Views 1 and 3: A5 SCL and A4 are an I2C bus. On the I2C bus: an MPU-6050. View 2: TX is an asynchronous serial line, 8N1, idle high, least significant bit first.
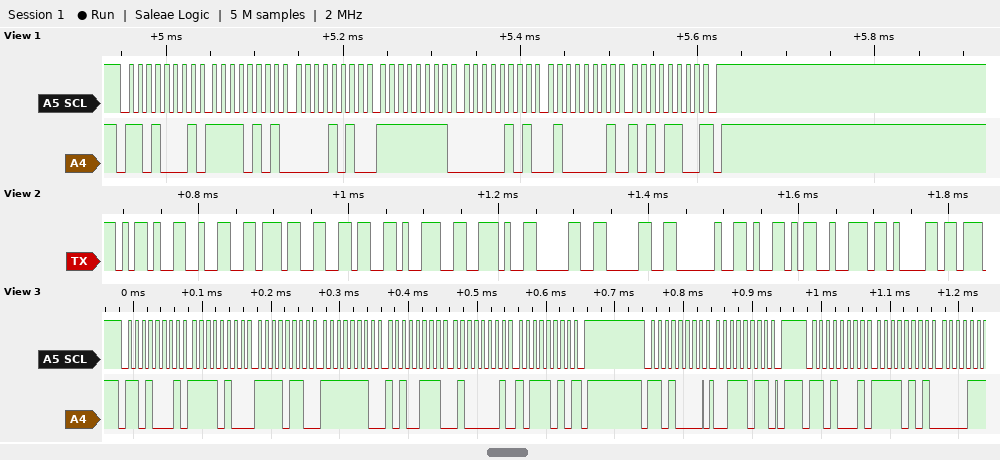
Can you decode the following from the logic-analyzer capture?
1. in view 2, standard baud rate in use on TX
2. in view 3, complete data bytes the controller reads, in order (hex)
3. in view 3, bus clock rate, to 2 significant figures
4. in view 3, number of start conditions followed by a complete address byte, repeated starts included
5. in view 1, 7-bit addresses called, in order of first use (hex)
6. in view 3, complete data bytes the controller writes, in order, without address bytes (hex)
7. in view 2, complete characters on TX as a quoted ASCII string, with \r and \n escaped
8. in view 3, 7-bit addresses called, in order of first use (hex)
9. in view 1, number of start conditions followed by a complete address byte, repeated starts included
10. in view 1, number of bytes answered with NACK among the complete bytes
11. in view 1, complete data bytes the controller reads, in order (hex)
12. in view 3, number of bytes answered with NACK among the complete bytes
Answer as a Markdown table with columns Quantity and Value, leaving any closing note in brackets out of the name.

| Quantity | Value |
|---|---|
| in view 2, standard baud rate in use on TX | 115200 baud |
| in view 3, complete data bytes the controller reads, in order | F4 F6 FE A7 41 BA F5 |
| in view 3, bus clock rate, to 2 significant figures | 100 kHz |
| in view 3, number of start conditions followed by a complete address byte, repeated starts included | 3 |
| in view 1, 7-bit addresses called, in order of first use | 0x68 |
| in view 3, complete data bytes the controller writes, in order, without address bytes | 3B |
| in view 2, complete characters on TX as a quoted ASCII string, with \r and \n escaped | "-2769.00 Yra" |
| in view 3, 7-bit addresses called, in order of first use | 0x68 |
| in view 1, number of start conditions followed by a complete address byte, repeated starts included | 1 |
| in view 1, number of bytes answered with NACK among the complete bytes | 1 |
| in view 1, complete data bytes the controller reads, in order | F5 0A FF 05 41 AC |
| in view 3, number of bytes answered with NACK among the complete bytes | 1 |
